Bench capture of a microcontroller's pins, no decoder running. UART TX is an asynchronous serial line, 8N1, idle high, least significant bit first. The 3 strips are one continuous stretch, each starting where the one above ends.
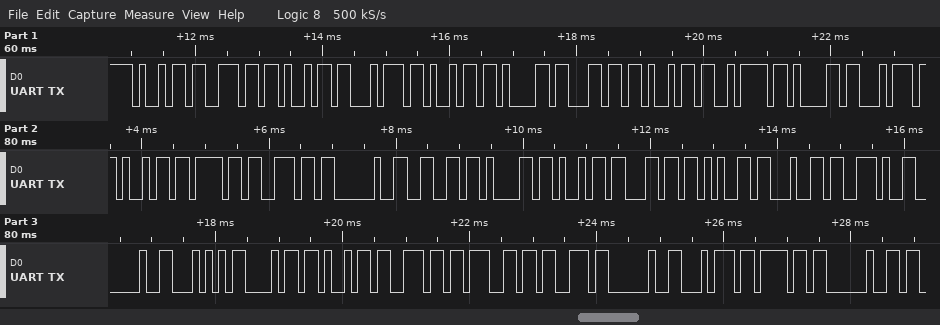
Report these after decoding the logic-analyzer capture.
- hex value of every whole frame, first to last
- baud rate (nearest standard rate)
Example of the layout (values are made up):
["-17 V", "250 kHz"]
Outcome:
["69 6E 69 74 69 61 6C 69 7A 61 74 69 6F 6E 20 66 61 69 6C 65 64 2E 20 54 68 69 6E 67 73 20 74 6F 20", "9600 baud"]
